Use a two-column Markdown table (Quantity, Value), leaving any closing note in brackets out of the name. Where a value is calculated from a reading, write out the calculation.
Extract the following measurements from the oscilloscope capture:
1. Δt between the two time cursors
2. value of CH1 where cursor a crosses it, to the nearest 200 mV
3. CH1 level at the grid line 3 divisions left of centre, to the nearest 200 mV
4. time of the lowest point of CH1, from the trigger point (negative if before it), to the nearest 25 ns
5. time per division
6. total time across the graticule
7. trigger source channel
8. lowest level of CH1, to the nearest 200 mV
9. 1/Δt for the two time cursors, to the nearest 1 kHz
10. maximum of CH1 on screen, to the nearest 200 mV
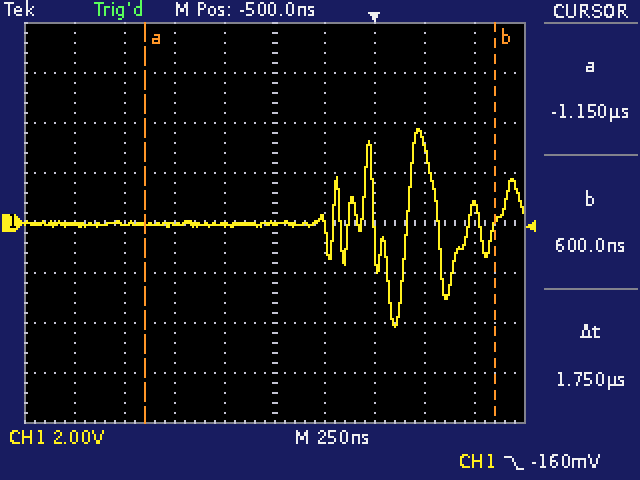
| Quantity | Value |
|---|---|
| Δt between the two time cursors | 1.75 µs |
| value of CH1 where cursor a crosses it, to the nearest 200 mV | 0.0 V |
| CH1 level at the grid line 3 divisions left of centre, to the nearest 200 mV | 0.0 V |
| time of the lowest point of CH1, from the trigger point (negative if before it), to the nearest 25 ns | +100 ns |
| time per division | 250 ns |
| total time across the graticule | 2.5 µs |
| trigger source channel | CH1 |
| lowest level of CH1, to the nearest 200 mV | -4.2 V |
| 1/Δt for the two time cursors, to the nearest 1 kHz | 1 / 1.75 µs ≈ 571 kHz |
| maximum of CH1 on screen, to the nearest 200 mV | 3.8 V |
